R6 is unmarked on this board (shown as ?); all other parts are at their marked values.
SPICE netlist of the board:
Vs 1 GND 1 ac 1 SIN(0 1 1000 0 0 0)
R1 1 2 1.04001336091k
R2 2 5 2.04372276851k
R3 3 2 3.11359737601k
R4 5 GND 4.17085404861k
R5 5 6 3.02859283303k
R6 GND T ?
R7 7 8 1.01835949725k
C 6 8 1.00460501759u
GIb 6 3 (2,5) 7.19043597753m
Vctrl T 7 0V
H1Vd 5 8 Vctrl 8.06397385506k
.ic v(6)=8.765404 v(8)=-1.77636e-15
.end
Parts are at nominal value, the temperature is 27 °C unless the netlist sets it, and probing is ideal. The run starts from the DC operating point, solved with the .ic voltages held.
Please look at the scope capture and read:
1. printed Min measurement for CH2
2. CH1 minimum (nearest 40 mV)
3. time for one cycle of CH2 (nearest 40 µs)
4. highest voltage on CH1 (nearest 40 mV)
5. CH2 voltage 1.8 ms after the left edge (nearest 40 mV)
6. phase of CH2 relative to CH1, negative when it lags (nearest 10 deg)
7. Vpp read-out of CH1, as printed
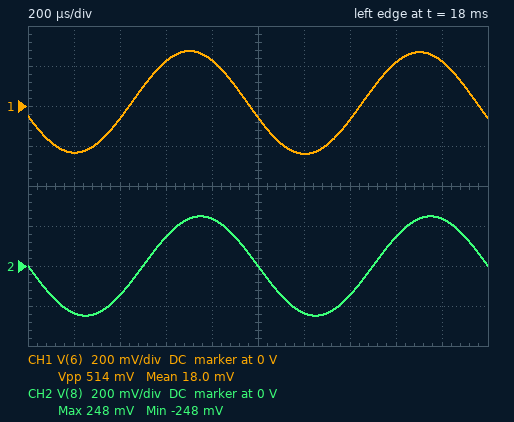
-248 mV
-240 mV
1.00 ms
280 mV
240 mV
-20 deg
514 mV
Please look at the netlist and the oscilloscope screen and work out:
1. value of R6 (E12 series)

680 Ω
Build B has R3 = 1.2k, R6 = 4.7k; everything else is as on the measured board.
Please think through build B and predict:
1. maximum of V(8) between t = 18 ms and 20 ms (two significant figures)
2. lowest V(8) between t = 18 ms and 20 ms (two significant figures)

2.9 V
-2.9 V
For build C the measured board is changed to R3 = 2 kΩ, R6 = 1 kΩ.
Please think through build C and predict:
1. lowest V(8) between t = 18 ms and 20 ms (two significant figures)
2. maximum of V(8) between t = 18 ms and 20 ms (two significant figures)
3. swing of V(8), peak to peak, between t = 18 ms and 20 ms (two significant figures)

-310 mV
310 mV
630 mV
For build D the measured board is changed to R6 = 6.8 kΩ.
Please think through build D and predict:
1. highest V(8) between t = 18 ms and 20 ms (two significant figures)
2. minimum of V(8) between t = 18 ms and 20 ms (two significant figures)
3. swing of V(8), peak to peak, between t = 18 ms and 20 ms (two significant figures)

13 V
-13 V
26 V
